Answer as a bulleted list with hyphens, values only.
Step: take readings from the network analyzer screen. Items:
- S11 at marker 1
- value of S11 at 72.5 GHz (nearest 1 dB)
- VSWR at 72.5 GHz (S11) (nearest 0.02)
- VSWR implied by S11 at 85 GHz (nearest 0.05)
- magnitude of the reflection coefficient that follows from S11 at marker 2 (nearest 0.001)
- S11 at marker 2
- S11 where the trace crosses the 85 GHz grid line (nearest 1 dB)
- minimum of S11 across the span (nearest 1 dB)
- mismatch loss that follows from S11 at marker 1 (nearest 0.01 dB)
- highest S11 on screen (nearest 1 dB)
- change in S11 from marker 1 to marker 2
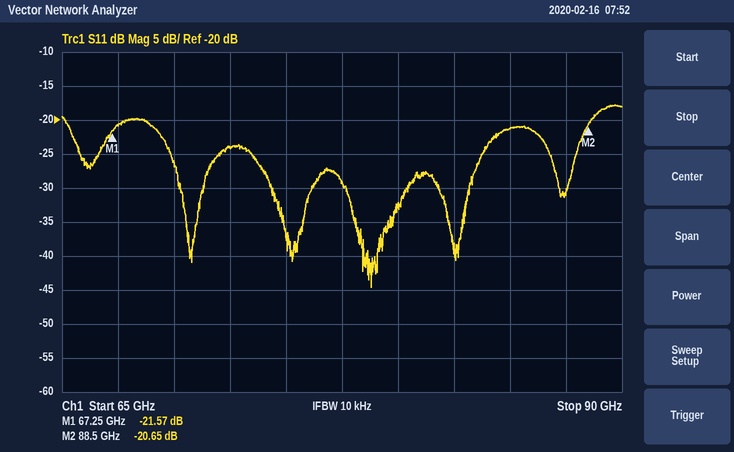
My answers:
- -21.57 dB
- -24 dB
- 1.14
- 1.20
- 0.093
- -20.65 dB
- -21 dB
- -45 dB
- 0.03 dB
- -18 dB
- 0.92 dB
